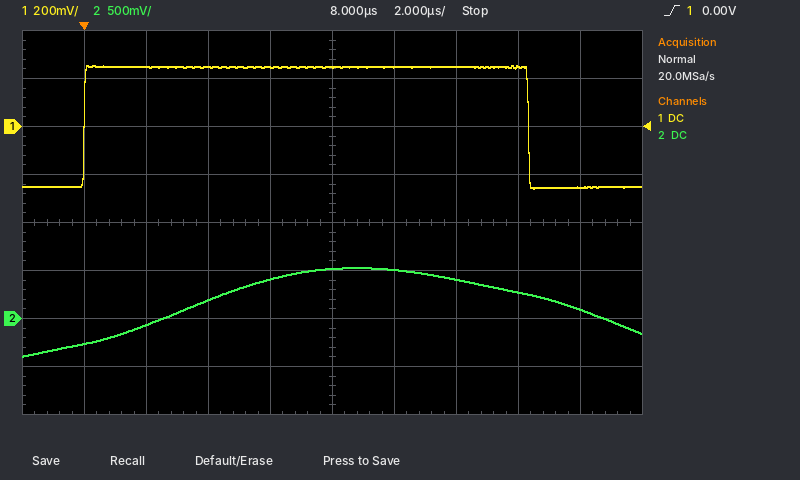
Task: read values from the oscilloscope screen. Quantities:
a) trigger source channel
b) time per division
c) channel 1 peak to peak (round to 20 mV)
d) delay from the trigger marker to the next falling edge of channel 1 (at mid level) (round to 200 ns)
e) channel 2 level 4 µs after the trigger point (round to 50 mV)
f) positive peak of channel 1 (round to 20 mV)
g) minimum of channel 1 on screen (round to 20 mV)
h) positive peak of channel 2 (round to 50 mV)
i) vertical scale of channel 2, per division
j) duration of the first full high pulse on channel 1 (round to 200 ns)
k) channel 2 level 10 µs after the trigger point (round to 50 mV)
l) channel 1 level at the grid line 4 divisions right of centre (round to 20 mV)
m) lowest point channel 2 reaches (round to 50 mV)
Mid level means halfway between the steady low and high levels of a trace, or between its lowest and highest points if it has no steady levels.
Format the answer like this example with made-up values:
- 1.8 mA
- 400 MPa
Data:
- channel 1
- 2 µs
- 520 mV
- 14.4 µs
- 200 mV
- 260 mV
- -260 mV
- 550 mV
- 500 mV
- 14.4 µs
- 500 mV
- -260 mV
- -400 mV
